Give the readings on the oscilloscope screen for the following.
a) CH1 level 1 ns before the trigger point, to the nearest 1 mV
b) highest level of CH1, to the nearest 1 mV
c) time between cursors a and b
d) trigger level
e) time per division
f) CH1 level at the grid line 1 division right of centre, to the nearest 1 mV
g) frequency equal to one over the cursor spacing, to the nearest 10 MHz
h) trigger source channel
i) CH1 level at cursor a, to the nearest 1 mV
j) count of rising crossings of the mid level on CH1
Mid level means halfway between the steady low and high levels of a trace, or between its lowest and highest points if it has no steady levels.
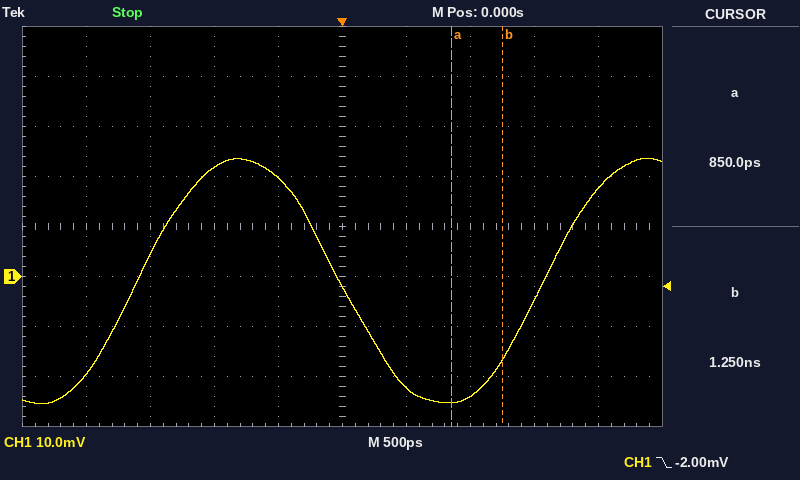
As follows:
22 mV
24 mV
400 ps
-2.00 mV
500 ps
-22 mV
2.50 GHz
CH1
-25 mV
2
